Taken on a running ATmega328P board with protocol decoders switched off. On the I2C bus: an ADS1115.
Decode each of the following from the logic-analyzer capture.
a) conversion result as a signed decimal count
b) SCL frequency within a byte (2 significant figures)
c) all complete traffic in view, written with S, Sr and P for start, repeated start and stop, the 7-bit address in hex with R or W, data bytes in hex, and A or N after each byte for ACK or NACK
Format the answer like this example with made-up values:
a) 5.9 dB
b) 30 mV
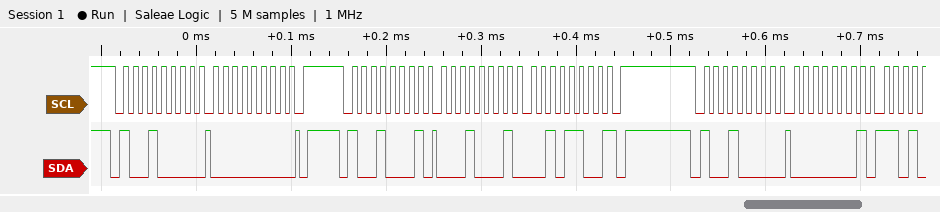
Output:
a) 4396
b) 100 kHz
c) S 48W A 00 A P S 48R A 11 A 2C N P S 48W A 01 A
